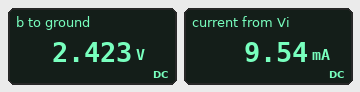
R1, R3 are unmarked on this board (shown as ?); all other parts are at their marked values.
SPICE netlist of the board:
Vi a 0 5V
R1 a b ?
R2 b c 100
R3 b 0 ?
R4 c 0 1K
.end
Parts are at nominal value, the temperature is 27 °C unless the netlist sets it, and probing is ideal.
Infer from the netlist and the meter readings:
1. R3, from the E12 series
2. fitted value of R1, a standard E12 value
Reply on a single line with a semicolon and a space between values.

330 Ω; 270 Ω
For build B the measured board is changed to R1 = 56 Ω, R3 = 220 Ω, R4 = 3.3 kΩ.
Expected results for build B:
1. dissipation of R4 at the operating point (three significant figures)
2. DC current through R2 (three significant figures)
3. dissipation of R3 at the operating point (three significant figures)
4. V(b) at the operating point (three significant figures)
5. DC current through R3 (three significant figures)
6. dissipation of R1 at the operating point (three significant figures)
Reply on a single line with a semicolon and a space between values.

4.42 mW; 1.16 mA; 70.3 mW; 3.93 V; 17.9 mA; 20.3 mW
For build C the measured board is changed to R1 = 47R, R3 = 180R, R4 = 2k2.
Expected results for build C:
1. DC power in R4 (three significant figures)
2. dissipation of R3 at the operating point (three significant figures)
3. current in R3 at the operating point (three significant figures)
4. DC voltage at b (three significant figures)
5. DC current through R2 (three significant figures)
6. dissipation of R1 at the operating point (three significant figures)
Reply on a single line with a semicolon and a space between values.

6.33 mW; 84.6 mW; 21.7 mA; 3.90 V; 1.70 mA; 25.7 mW
